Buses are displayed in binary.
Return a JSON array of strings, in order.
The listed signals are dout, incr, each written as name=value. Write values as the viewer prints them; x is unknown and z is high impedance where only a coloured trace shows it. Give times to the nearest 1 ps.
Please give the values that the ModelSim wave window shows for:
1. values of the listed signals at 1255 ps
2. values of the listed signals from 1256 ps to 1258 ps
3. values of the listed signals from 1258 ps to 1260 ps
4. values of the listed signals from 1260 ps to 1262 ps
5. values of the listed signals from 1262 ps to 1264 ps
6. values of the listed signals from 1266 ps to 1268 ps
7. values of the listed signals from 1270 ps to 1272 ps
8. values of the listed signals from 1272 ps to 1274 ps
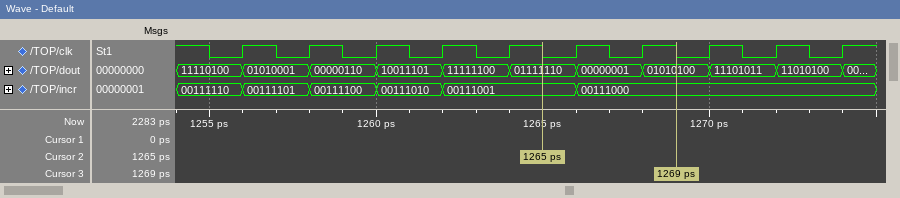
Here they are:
["dout=11110100, incr=00111110", "dout=01010001, incr=00111101", "dout=00000110, incr=00111100", "dout=10011101, incr=00111010", "dout=11111100, incr=00111001", "dout=00000001, incr=00111000", "dout=11101011, incr=00111000", "dout=11010100, incr=00111000"]
